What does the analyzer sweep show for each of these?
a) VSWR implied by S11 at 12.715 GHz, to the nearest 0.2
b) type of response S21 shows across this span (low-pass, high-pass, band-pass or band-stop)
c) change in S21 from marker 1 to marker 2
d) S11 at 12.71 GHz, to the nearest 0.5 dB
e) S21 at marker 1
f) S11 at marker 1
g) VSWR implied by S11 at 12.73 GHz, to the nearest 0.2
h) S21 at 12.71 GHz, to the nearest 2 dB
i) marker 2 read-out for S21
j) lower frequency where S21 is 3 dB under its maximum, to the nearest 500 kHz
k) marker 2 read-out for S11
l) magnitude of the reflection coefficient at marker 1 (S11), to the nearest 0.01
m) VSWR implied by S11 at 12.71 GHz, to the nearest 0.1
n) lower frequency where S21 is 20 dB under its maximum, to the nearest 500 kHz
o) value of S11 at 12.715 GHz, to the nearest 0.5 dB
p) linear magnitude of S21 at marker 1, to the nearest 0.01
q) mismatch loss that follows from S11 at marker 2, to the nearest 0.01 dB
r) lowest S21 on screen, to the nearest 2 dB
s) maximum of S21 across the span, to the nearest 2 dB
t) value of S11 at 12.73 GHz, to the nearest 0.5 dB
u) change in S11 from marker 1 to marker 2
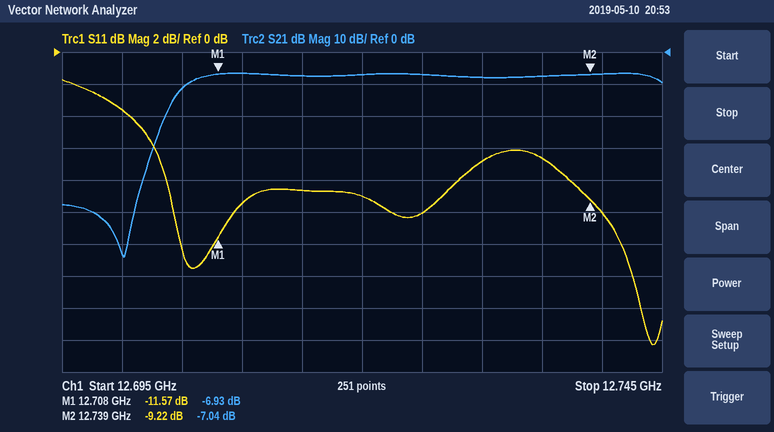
2.2
high-pass
-0.11 dB
-9.5 dB
-6.93 dB
-11.57 dB
2.6
-6 dB
-7.04 dB
12.7055 GHz
-9.22 dB
0.26
2.0
12.7030 GHz
-8.5 dB
0.45
0.55 dB
-64 dB
-6 dB
-7.0 dB
2.35 dB
